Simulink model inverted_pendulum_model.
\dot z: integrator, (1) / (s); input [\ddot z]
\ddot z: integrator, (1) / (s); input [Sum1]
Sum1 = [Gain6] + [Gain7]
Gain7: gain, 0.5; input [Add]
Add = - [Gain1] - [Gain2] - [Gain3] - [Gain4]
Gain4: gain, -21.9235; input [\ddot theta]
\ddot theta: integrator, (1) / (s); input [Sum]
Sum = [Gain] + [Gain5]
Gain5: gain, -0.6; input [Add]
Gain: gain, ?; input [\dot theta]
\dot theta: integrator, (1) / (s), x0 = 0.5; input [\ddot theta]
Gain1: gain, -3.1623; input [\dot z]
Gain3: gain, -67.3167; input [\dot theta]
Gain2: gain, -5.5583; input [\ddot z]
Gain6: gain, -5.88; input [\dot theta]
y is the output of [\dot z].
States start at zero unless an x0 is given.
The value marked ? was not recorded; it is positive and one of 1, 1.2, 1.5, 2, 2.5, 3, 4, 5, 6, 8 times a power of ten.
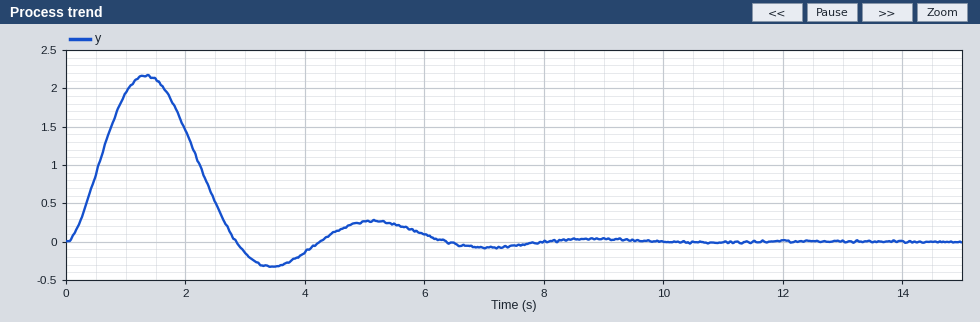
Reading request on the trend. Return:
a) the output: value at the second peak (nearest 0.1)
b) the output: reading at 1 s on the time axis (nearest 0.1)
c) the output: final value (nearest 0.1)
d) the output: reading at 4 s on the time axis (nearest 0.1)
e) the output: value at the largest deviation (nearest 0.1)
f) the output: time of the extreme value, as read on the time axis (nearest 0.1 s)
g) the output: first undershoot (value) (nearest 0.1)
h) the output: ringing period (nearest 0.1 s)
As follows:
0.3
1.9
0.0
-0.1
2.2
1.3 s
-0.3
3.8 s
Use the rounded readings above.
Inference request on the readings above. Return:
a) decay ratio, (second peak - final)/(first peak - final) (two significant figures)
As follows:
0.14
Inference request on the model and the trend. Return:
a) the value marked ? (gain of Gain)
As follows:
20
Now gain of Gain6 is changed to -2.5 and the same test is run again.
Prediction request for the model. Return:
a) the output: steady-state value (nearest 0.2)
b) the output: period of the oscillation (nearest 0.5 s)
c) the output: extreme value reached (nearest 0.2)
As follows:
0.0
3.0 s
2.4
